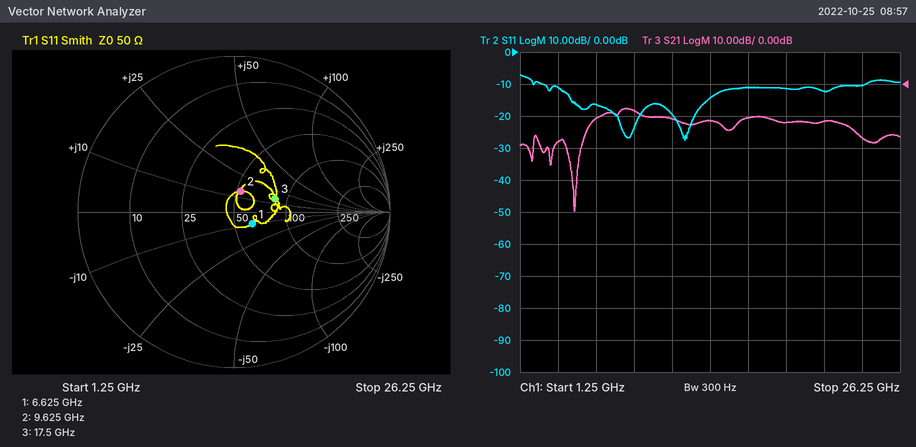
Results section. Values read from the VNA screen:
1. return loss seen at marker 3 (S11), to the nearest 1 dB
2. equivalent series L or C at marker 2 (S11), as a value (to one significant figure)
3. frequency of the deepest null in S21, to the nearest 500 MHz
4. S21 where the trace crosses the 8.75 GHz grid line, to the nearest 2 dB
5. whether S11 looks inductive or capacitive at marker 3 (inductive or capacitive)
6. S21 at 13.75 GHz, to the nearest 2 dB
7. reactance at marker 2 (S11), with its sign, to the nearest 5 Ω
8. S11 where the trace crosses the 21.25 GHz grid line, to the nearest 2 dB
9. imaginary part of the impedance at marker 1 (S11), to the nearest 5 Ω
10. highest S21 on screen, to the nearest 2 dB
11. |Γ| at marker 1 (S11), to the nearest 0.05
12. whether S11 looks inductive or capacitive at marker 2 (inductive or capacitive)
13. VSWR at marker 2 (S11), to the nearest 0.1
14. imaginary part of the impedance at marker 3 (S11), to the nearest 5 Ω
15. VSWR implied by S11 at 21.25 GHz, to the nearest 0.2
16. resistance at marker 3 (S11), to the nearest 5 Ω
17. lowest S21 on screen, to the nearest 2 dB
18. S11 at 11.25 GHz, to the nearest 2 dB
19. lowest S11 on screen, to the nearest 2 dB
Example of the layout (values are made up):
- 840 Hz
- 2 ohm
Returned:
- 11 dB
- 200 pH
- 5.0 GHz
- -8 dB
- inductive
- -12 dB
- +15 Ω
- -12 dB
- -10 Ω
- -8 dB
- 0.15
- inductive
- 1.3
- +15 Ω
- 1.6
- 85 Ω
- -40 dB
- -20 dB
- -28 dB
